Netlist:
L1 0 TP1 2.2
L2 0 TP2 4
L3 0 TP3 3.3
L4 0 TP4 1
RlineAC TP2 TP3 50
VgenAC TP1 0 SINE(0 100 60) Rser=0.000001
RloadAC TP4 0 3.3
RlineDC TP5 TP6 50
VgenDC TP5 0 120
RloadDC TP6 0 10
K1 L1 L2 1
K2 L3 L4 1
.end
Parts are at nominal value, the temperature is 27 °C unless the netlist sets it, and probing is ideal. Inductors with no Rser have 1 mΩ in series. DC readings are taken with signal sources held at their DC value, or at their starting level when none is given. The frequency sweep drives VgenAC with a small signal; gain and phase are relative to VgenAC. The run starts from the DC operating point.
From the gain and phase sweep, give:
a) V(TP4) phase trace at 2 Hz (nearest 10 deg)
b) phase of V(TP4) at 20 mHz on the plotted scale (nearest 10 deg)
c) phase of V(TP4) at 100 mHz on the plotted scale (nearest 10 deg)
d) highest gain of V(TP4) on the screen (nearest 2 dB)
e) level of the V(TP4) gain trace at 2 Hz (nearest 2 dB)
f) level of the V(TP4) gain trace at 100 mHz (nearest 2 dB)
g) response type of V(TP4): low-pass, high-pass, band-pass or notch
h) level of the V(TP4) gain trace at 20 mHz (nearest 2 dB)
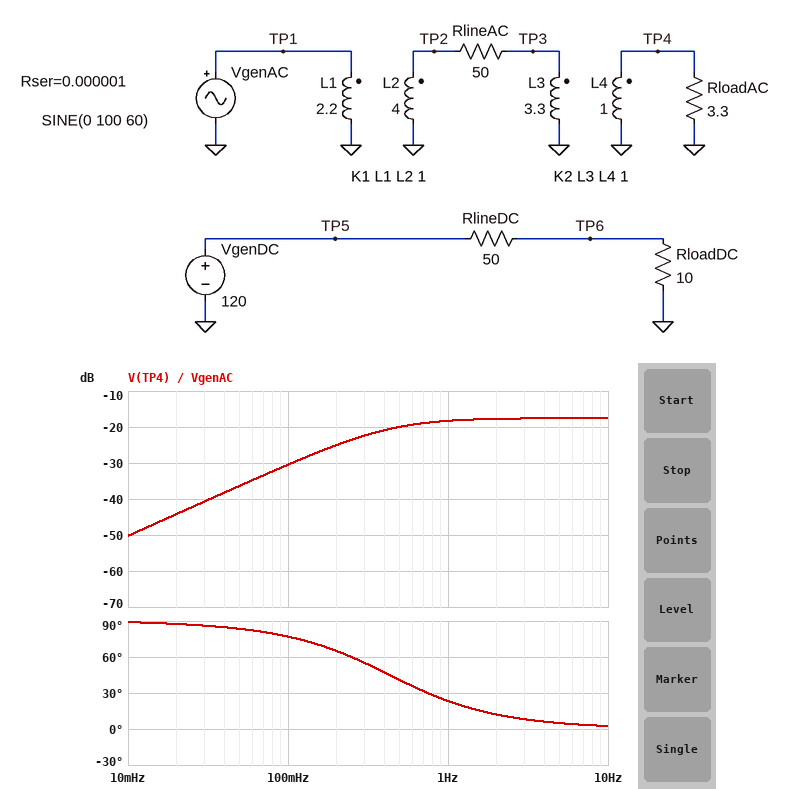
10 deg
90 deg
80 deg
-18 dB
-18 dB
-30 dB
high-pass
-44 dB
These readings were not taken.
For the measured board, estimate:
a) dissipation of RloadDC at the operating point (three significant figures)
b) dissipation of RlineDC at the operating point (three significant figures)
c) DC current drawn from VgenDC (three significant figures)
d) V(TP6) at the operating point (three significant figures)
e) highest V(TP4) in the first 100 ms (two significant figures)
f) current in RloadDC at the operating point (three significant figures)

40.0 W
200 W
2.00 A
20.0 V
13 V
2.00 A
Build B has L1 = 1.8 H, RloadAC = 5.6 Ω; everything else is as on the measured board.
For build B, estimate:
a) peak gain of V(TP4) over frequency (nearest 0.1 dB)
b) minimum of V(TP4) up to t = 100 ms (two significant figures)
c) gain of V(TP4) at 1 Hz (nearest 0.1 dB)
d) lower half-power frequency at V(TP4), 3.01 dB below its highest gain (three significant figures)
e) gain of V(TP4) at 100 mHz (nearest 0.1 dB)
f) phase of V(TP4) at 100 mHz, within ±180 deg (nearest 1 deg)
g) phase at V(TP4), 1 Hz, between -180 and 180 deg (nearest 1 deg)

-13.1 dB
-22 V
-14.6 dB
651 mHz
-29.5 dB
81 deg
33 deg
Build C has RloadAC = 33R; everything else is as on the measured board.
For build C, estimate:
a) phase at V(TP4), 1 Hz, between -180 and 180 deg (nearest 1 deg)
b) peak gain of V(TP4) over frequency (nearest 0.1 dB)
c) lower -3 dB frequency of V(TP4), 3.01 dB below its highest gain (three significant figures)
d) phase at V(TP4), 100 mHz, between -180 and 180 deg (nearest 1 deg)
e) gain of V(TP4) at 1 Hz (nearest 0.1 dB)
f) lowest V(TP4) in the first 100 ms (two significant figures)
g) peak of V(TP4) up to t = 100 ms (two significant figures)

59 deg
-5.9 dB
1.65 Hz
87 deg
-11.6 dB
-52 V
50 V
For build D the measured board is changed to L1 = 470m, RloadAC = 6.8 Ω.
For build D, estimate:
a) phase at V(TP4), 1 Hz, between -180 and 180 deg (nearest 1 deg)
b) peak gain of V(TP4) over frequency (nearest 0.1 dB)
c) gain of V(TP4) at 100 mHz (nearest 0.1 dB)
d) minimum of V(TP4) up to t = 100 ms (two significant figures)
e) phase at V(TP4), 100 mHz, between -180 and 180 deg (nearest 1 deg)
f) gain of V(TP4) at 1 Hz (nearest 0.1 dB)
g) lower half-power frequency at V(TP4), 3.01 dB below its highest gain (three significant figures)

37 deg
-6.1 dB
-23.6 dB
-50 V
83 deg
-8.0 dB
747 mHz
